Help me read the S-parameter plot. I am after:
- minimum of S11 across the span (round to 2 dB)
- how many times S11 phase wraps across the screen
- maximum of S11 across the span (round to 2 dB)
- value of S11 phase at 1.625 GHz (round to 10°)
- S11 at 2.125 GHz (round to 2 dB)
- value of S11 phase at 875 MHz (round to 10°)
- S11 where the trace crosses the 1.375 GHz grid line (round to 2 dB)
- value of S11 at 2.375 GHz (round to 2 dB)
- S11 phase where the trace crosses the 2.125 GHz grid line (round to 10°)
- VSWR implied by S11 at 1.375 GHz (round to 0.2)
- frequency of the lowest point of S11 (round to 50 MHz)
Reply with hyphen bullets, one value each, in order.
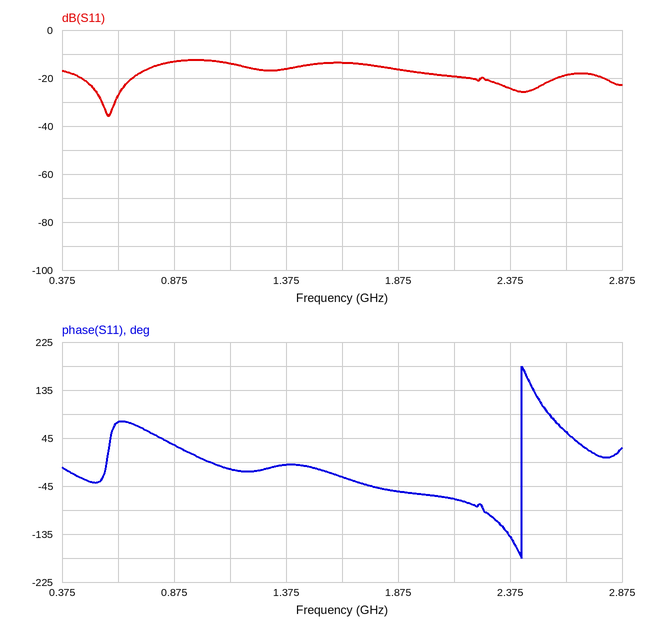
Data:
- -36 dB
- 1
- -12 dB
- -30°
- -20 dB
- 30°
- -16 dB
- -24 dB
- -70°
- 1.4
- 600 MHz
